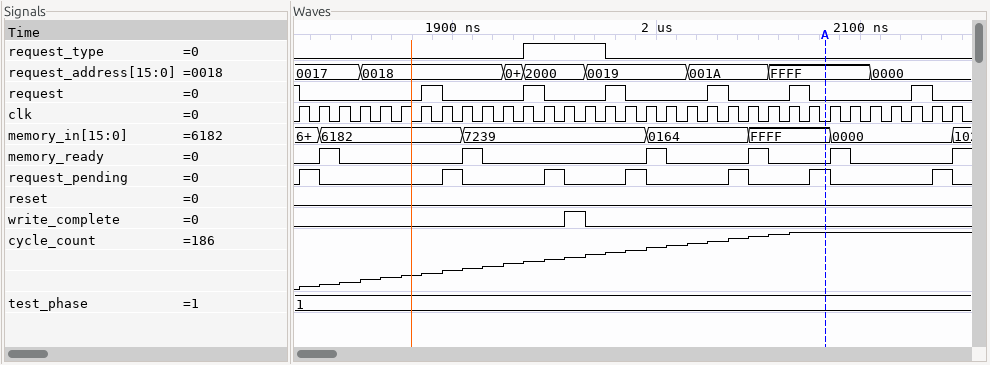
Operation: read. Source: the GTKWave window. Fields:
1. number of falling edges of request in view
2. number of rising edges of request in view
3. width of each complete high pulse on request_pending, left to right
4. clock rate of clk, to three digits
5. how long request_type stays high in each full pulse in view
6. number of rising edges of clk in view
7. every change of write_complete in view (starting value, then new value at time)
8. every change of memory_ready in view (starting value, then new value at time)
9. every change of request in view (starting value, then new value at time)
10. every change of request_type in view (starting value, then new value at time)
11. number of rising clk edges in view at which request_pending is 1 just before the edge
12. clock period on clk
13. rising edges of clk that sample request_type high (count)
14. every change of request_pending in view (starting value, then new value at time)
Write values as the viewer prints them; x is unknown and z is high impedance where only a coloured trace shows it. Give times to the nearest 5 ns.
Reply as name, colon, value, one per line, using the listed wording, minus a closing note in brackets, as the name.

number of falling edges of request in view: 7
number of rising edges of request in view: 6
width of each complete high pulse on request_pending, left to right: 10 ns, 10 ns, 10 ns, 10 ns, 10 ns, 10 ns, 10 ns
clock rate of clk, to three digits: 100 MHz
how long request_type stays high in each full pulse in view: 40 ns
number of rising edges of clk in view: 33
every change of write_complete in view: 0, 1 at 1955 ns, 0 at 1965 ns
every change of memory_ready in view: 0, 1 at 1835 ns, 0 at 1845 ns, 1 at 1905 ns, 0 at 1915 ns, 1 at 1995 ns, 0 at 2005 ns, 1 at 2045 ns, 0 at 2055 ns, 1 at 2085 ns, 0 at 2095 ns, 1 at 2145 ns
every change of request in view: 1, 0 at 1825 ns, 1 at 1885 ns, 0 at 1895 ns, 1 at 1935 ns, 0 at 1945 ns, 1 at 1975 ns, 0 at 1985 ns, 1 at 2025 ns, 0 at 2035 ns, 1 at 2065 ns, 0 at 2075 ns, 1 at 2125 ns, 0 at 2135 ns
every change of request_type in view: 0, 1 at 1935 ns, 0 at 1975 ns
number of rising clk edges in view at which request_pending is 1 just before the edge: 7
clock period on clk: 10 ns
rising edges of clk that sample request_type high: 4
every change of request_pending in view: 0, 1 at 1825 ns, 0 at 1835 ns, 1 at 1895 ns, 0 at 1905 ns, 1 at 1945 ns, 0 at 1955 ns, 1 at 1985 ns, 0 at 1995 ns, 1 at 2035 ns, 0 at 2045 ns, 1 at 2075 ns, 0 at 2085 ns, 1 at 2135 ns, 0 at 2145 ns
